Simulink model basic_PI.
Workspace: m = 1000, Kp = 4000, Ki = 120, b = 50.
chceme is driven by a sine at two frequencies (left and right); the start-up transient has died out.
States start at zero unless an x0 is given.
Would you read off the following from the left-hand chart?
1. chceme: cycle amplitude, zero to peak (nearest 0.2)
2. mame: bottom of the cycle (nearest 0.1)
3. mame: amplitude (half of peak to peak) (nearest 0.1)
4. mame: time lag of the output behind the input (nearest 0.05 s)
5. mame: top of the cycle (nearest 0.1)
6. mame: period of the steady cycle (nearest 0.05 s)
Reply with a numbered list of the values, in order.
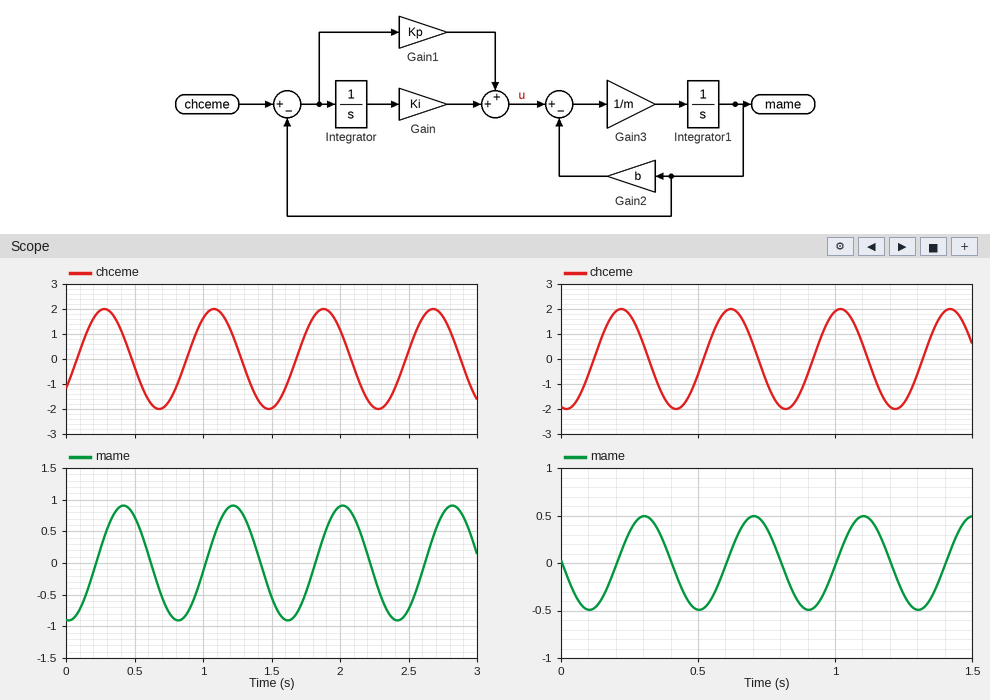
1. 2.0
2. -0.9
3. 0.9
4. 0.15 s
5. 0.9
6. 0.80 s
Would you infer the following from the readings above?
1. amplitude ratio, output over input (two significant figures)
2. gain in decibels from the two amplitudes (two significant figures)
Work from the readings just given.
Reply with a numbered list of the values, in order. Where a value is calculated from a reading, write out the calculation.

1. 0.9 / 2 = 0.45
2. 20 log10(0.9 / 2) = -6.9 dB
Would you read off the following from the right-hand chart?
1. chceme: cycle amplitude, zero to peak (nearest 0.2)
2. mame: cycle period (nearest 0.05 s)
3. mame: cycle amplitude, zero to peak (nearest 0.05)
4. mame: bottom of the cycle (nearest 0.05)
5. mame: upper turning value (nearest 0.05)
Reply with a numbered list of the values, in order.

1. 2.0
2. 0.40 s
3. 0.50
4. -0.50
5. 0.50
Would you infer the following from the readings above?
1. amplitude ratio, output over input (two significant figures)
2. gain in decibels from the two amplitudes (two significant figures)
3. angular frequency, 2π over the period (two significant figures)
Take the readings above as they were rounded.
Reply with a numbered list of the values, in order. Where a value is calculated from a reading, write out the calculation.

1. 0.5 / 2 = 0.25
2. 20 log10(0.5 / 2) = -12 dB
3. 2π / 0.4 = 16 rad/s
